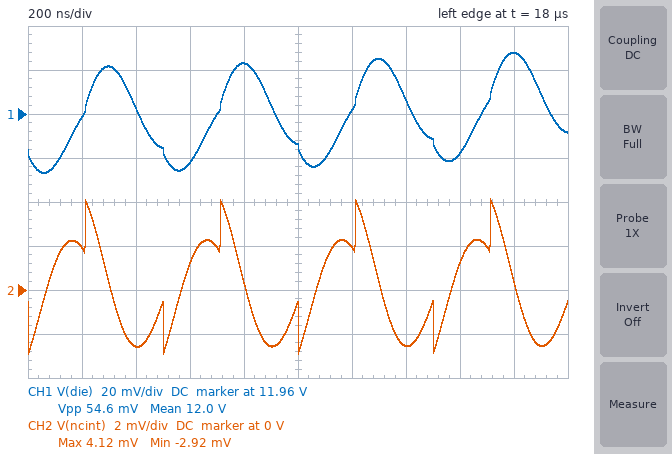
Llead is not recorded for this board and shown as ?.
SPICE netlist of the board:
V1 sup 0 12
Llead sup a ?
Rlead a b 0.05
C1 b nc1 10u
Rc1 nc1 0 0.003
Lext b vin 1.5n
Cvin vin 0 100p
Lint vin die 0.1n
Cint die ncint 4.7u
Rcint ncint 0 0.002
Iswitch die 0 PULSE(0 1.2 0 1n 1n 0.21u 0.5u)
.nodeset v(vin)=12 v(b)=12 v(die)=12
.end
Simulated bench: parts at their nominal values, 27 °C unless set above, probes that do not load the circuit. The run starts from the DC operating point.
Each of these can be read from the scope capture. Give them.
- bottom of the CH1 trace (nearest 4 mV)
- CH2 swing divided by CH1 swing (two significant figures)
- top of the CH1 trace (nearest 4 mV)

11.932 V
0.13
11.988 V
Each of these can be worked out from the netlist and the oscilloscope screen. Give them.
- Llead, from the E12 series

330 nH
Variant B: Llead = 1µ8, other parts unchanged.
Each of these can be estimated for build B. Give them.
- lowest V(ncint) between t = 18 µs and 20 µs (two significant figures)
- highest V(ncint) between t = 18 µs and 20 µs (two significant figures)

-2.7 mV
4.3 mV
